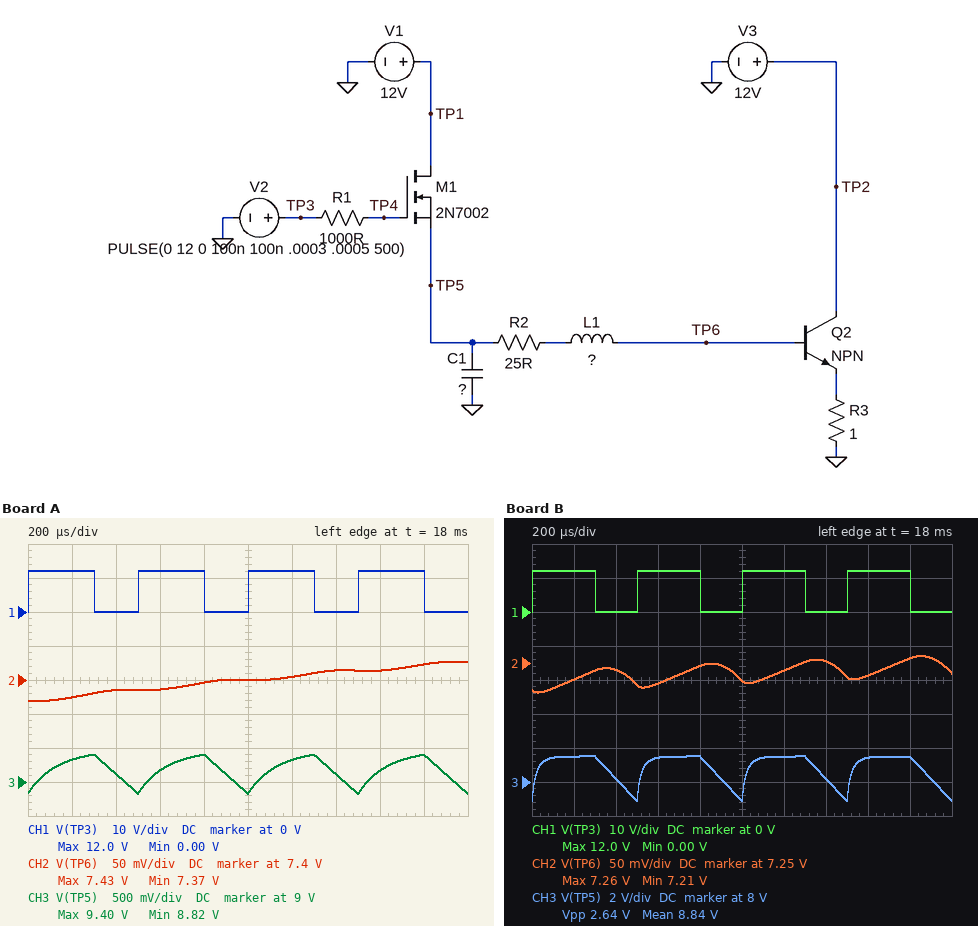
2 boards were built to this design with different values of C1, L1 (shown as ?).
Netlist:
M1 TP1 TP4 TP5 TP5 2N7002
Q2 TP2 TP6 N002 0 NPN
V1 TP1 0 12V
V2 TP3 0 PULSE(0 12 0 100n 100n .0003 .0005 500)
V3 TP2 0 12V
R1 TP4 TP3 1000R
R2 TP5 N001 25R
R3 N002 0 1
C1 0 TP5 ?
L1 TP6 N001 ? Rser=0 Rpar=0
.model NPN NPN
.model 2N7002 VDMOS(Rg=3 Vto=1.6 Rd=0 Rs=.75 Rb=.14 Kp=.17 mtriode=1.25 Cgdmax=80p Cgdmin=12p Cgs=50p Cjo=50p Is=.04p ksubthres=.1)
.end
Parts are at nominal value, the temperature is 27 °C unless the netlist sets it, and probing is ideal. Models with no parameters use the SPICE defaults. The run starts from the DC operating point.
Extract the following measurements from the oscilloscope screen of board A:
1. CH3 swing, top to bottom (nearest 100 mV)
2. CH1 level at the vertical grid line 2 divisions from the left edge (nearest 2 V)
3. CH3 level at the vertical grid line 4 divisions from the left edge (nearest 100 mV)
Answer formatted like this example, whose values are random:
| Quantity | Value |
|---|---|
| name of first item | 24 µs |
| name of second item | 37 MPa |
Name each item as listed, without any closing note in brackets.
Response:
| Quantity | Value |
|---|---|
| CH3 swing, top to bottom | 600 mV |
| CH1 level at the vertical grid line 2 divisions from the left edge | 0 V |
| CH3 level at the vertical grid line 4 divisions from the left edge | 9.4 V |
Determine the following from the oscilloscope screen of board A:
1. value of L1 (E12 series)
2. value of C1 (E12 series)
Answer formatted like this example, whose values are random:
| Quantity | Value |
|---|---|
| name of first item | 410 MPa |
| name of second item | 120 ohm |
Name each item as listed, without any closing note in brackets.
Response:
| Quantity | Value |
|---|---|
| value of L1 | 680 mH |
| value of C1 | 22 µF |
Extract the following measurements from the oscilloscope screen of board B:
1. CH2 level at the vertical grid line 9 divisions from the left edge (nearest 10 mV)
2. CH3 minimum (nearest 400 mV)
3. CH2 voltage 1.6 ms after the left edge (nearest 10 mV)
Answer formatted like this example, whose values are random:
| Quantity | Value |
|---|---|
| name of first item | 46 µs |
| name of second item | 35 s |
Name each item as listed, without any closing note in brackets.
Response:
| Quantity | Value |
|---|---|
| CH2 level at the vertical grid line 9 divisions from the left edge | 7.26 V |
| CH3 minimum | 6.8 V |
| CH2 voltage 1.6 ms after the left edge | 7.23 V |
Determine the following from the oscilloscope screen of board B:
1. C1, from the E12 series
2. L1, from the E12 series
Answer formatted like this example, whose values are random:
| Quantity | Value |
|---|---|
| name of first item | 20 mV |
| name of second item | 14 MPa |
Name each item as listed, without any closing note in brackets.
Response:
| Quantity | Value |
|---|---|
| C1, from the E12 series | 4.7 µF |
| L1, from the E12 series | 560 mH |
